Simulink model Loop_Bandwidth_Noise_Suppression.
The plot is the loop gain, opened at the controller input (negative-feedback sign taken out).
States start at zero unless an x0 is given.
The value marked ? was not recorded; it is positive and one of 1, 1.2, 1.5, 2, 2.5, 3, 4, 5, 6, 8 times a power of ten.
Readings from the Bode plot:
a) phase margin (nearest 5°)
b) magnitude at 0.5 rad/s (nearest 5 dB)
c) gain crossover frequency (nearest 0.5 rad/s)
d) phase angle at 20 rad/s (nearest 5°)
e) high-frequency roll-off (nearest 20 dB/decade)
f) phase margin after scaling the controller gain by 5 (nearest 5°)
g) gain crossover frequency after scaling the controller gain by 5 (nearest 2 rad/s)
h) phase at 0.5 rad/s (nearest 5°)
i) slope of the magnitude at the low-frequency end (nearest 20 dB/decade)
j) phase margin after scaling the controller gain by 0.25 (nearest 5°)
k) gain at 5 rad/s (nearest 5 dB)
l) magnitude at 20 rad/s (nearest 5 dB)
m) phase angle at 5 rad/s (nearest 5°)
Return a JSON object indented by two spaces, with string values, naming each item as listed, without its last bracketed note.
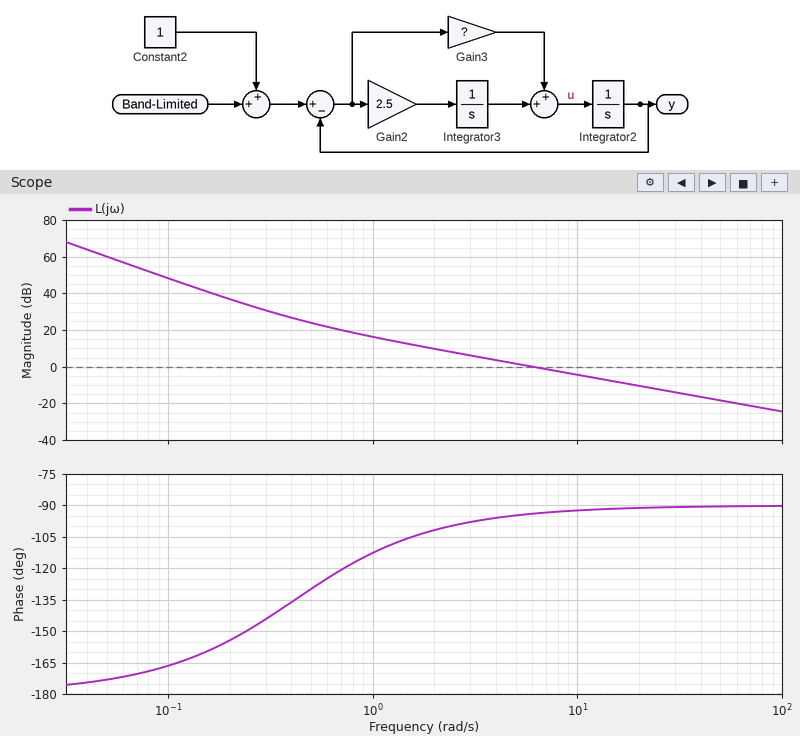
{
  "phase margin": "85°",
  "magnitude at 0.5 rad/s": "25 dB",
  "gain crossover frequency": "6.0 rad/s",
  "phase angle at 20 rad/s": "-90°",
  "high-frequency roll-off": "-20 dB/decade",
  "phase margin after scaling the controller gain by 5": "90°",
  "gain crossover frequency after scaling the controller gain by 5": "30 rad/s",
  "phase at 0.5 rad/s": "-130°",
  "slope of the magnitude at the low-frequency end": "-40 dB/decade",
  "phase margin after scaling the controller gain by 0.25": "75°",
  "gain at 5 rad/s": "0 dB",
  "magnitude at 20 rad/s": "-10 dB",
  "phase angle at 5 rad/s": "-95°"
}
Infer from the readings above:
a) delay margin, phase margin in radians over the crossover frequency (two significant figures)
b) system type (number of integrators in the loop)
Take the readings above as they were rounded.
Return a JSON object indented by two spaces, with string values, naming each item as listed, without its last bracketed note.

{
  "delay margin, phase margin in radians over the crossover frequency": "0.25 s",
  "system type": "2"
}
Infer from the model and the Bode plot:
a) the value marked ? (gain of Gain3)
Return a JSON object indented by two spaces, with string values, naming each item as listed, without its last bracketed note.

{
  "the value marked ?": "6"
}
